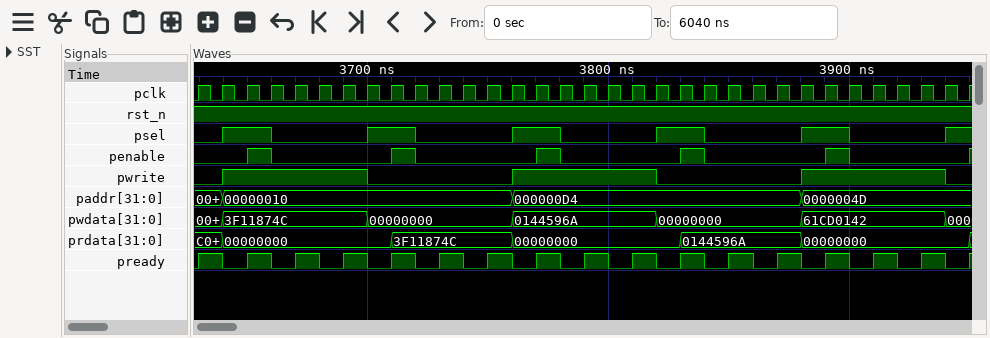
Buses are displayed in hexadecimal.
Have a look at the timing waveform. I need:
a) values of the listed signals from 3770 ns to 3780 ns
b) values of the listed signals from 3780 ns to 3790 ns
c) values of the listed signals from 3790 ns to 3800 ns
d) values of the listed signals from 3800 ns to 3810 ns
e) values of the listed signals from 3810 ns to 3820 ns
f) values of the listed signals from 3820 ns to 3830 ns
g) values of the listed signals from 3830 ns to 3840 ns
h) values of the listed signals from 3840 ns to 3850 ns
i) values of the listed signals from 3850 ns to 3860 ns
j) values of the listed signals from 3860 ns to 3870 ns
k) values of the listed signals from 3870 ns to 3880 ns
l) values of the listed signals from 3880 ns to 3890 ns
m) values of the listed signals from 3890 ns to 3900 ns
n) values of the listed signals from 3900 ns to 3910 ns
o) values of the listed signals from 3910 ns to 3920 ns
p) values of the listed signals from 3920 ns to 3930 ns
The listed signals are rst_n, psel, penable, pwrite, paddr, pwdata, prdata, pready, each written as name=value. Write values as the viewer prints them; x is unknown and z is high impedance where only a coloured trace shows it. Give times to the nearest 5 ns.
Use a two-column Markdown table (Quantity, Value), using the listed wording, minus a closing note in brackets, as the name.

| Quantity | Value |
|---|---|
| values of the listed signals from 3770 ns to 3780 ns | rst_n=1, psel=1, penable=1, pwrite=1, paddr=000000D4, pwdata=0144596A, prdata=00000000, pready=1 |
| values of the listed signals from 3780 ns to 3790 ns | rst_n=1, psel=0, penable=0, pwrite=1, paddr=000000D4, pwdata=0144596A, prdata=00000000, pready=0 |
| values of the listed signals from 3790 ns to 3800 ns | rst_n=1, psel=0, penable=0, pwrite=1, paddr=000000D4, pwdata=0144596A, prdata=00000000, pready=1 |
| values of the listed signals from 3800 ns to 3810 ns | rst_n=1, psel=0, penable=0, pwrite=1, paddr=000000D4, pwdata=0144596A, prdata=00000000, pready=0 |
| values of the listed signals from 3810 ns to 3820 ns | rst_n=1, psel=0, penable=0, pwrite=1, paddr=000000D4, pwdata=0144596A, prdata=00000000, pready=1 |
| values of the listed signals from 3820 ns to 3830 ns | rst_n=1, psel=1, penable=0, pwrite=0, paddr=000000D4, pwdata=00000000, prdata=00000000, pready=0 |
| values of the listed signals from 3830 ns to 3840 ns | rst_n=1, psel=1, penable=1, pwrite=0, paddr=000000D4, pwdata=00000000, prdata=0144596A, pready=1 |
| values of the listed signals from 3840 ns to 3850 ns | rst_n=1, psel=0, penable=0, pwrite=0, paddr=000000D4, pwdata=00000000, prdata=0144596A, pready=0 |
| values of the listed signals from 3850 ns to 3860 ns | rst_n=1, psel=0, penable=0, pwrite=0, paddr=000000D4, pwdata=00000000, prdata=0144596A, pready=1 |
| values of the listed signals from 3860 ns to 3870 ns | rst_n=1, psel=0, penable=0, pwrite=0, paddr=000000D4, pwdata=00000000, prdata=0144596A, pready=0 |
| values of the listed signals from 3870 ns to 3880 ns | rst_n=1, psel=0, penable=0, pwrite=0, paddr=000000D4, pwdata=00000000, prdata=0144596A, pready=1 |
| values of the listed signals from 3880 ns to 3890 ns | rst_n=1, psel=1, penable=0, pwrite=1, paddr=0000004D, pwdata=61CD0142, prdata=00000000, pready=0 |
| values of the listed signals from 3890 ns to 3900 ns | rst_n=1, psel=1, penable=1, pwrite=1, paddr=0000004D, pwdata=61CD0142, prdata=00000000, pready=1 |
| values of the listed signals from 3900 ns to 3910 ns | rst_n=1, psel=0, penable=0, pwrite=1, paddr=0000004D, pwdata=61CD0142, prdata=00000000, pready=0 |
| values of the listed signals from 3910 ns to 3920 ns | rst_n=1, psel=0, penable=0, pwrite=1, paddr=0000004D, pwdata=61CD0142, prdata=00000000, pready=1 |
| values of the listed signals from 3920 ns to 3930 ns | rst_n=1, psel=0, penable=0, pwrite=1, paddr=0000004D, pwdata=61CD0142, prdata=00000000, pready=0 |
